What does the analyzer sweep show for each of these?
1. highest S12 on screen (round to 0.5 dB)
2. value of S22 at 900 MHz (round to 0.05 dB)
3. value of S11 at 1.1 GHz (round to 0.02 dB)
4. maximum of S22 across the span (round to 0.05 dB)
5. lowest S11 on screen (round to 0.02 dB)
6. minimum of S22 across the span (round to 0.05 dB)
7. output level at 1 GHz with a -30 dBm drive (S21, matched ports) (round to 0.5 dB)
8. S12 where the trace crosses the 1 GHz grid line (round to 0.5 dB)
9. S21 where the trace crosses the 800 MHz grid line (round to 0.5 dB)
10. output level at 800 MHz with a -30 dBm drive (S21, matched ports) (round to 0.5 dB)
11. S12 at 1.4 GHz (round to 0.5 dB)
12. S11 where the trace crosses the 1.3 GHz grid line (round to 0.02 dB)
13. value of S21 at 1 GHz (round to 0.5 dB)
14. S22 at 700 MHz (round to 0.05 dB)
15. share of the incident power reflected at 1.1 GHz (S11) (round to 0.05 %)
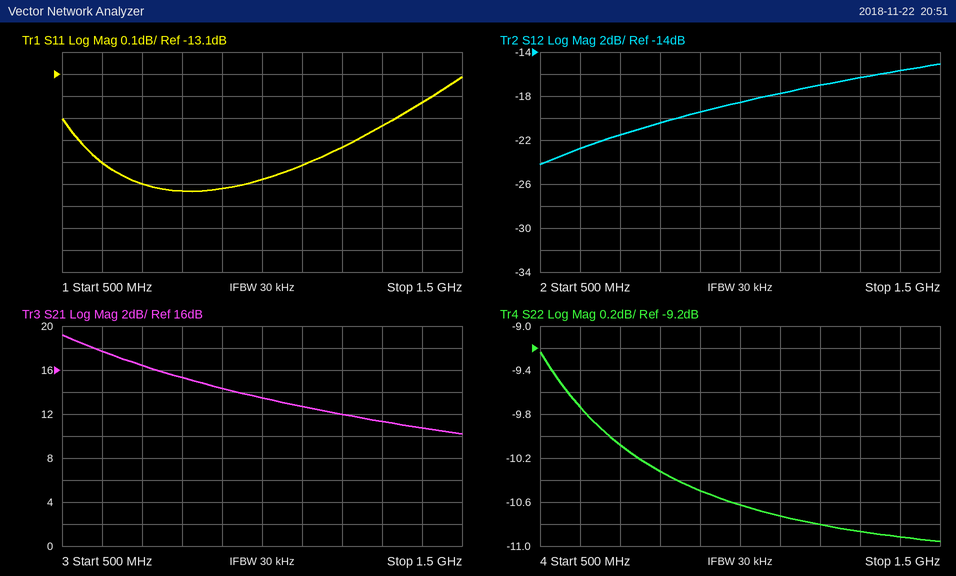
-15.0 dB
-10.50 dB
-13.52 dB
-9.25 dB
-13.64 dB
-10.95 dB
-16.5 dBm
-18.5 dB
15.5 dB
-14.5 dBm
-15.5 dB
-13.34 dB
13.5 dB
-10.10 dB
4.45 %
